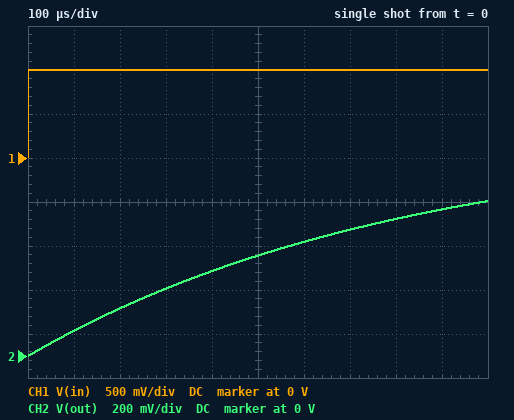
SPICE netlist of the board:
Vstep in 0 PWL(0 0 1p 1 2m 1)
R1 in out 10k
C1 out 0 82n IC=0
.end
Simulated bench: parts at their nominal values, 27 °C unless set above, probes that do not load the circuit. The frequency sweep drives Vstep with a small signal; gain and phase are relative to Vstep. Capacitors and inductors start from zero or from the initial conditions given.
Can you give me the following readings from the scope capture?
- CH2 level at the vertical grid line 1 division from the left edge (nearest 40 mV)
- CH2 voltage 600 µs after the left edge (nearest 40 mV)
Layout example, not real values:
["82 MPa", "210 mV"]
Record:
["120 mV", "520 mV"]
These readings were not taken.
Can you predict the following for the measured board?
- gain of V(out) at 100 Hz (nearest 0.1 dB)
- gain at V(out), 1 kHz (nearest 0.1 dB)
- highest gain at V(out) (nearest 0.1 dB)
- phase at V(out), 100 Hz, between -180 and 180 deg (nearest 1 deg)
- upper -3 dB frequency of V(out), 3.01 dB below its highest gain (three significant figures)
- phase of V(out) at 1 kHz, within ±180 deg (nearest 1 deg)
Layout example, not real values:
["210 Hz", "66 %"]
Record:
["-1.0 dB", "-14.4 dB", "0 dB", "-27 deg", "194 Hz", "-79 deg"]
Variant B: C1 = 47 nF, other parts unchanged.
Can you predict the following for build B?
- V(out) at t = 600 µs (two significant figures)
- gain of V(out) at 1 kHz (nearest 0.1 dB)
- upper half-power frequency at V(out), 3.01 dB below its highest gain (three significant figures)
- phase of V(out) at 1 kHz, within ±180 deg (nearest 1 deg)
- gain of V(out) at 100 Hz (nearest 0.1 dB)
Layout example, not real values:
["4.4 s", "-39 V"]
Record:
["720 mV", "-9.9 dB", "339 Hz", "-71 deg", "-0.4 dB"]
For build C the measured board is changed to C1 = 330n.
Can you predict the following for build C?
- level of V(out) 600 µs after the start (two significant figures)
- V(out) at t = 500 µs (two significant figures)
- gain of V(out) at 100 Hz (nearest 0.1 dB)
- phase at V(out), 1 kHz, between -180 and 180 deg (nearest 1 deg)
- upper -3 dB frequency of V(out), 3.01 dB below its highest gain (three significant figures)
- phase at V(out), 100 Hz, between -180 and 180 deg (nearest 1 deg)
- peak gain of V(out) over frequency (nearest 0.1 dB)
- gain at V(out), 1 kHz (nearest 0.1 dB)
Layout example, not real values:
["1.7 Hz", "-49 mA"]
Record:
["170 mV", "140 mV", "-7.2 dB", "-87 deg", "48.2 Hz", "-64 deg", "0 dB", "-26.3 dB"]
